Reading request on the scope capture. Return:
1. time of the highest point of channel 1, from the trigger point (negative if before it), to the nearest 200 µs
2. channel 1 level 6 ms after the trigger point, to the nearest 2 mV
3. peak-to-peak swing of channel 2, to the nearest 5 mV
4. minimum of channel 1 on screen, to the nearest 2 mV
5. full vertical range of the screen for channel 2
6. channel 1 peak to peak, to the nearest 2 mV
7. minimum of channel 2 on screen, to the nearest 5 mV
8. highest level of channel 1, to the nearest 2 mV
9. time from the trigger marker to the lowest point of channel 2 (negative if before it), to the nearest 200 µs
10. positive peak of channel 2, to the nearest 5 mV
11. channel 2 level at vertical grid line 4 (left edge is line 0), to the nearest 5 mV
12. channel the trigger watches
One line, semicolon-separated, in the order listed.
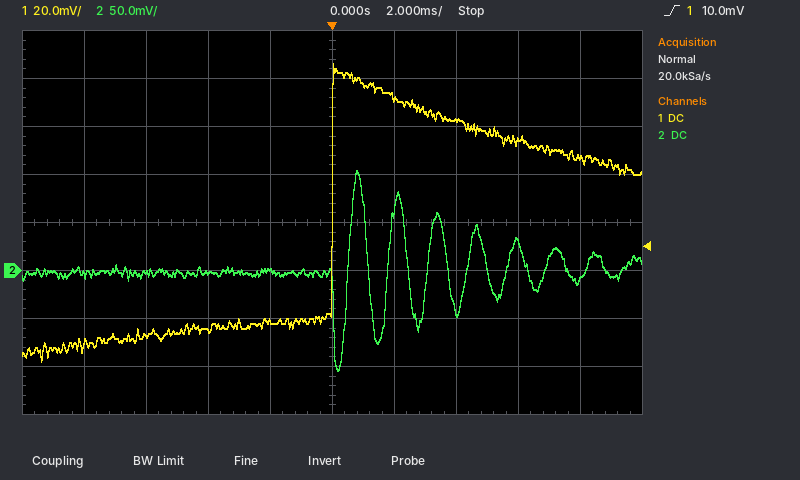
0.0 ms; 54 mV; 210 mV; -38 mV; 400 mV; 124 mV; -105 mV; 86 mV; +200 µs; 105 mV; 0 mV; channel 1
